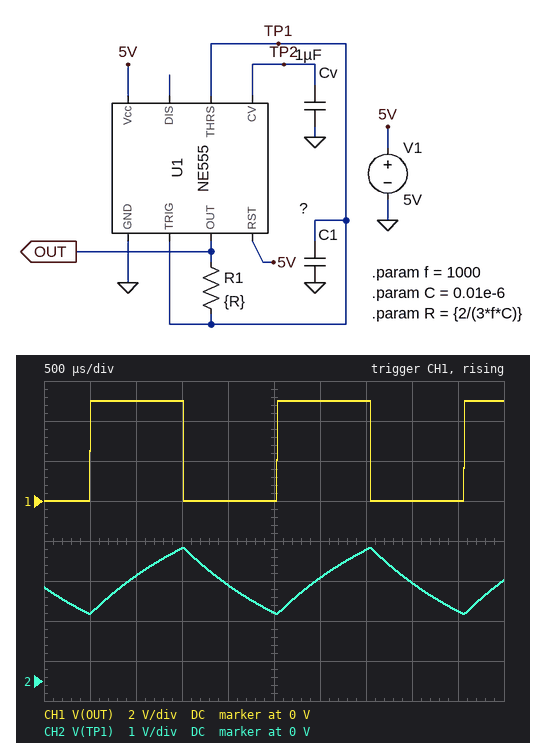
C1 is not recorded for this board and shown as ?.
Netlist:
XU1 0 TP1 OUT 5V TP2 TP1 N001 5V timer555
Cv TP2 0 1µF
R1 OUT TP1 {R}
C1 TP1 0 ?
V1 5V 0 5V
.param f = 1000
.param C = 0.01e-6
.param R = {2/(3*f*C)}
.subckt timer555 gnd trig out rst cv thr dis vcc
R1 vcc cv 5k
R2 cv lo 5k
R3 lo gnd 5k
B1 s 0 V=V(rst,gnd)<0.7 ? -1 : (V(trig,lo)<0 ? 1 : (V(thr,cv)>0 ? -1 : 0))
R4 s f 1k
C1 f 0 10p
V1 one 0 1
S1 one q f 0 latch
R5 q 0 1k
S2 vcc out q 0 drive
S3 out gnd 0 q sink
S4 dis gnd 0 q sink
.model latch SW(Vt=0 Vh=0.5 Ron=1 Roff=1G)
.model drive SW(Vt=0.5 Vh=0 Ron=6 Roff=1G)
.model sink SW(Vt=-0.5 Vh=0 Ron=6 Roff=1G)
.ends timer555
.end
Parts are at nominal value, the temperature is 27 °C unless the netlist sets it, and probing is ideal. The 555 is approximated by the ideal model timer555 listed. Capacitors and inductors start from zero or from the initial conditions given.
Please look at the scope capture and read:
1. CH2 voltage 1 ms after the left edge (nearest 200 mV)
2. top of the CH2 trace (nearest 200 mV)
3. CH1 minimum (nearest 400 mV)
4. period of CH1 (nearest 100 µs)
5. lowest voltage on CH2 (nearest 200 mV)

2.6 V
3.4 V
0 V
2.0 ms
1.6 V
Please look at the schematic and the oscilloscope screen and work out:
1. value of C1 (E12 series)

22 nF
